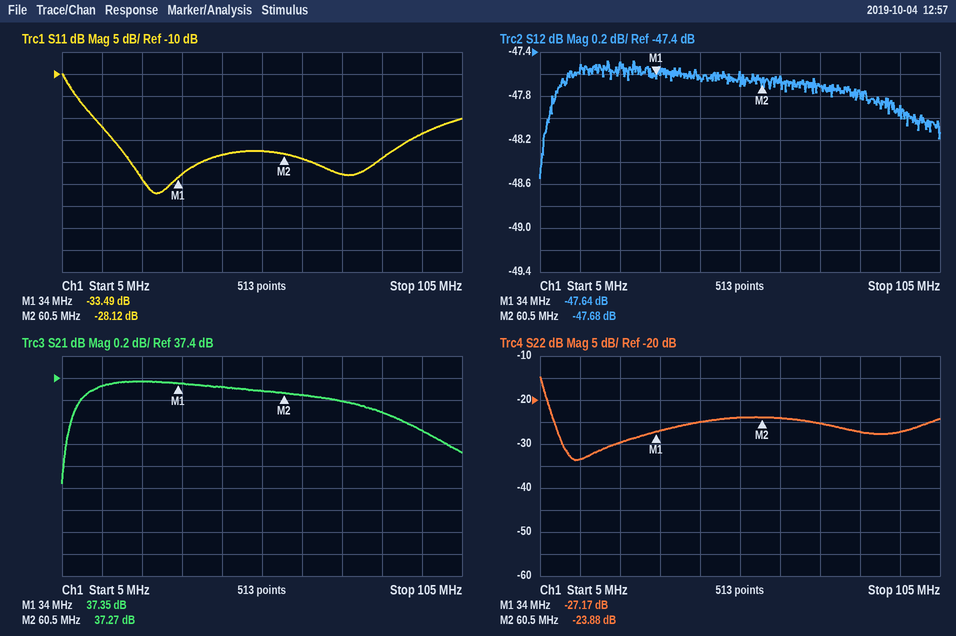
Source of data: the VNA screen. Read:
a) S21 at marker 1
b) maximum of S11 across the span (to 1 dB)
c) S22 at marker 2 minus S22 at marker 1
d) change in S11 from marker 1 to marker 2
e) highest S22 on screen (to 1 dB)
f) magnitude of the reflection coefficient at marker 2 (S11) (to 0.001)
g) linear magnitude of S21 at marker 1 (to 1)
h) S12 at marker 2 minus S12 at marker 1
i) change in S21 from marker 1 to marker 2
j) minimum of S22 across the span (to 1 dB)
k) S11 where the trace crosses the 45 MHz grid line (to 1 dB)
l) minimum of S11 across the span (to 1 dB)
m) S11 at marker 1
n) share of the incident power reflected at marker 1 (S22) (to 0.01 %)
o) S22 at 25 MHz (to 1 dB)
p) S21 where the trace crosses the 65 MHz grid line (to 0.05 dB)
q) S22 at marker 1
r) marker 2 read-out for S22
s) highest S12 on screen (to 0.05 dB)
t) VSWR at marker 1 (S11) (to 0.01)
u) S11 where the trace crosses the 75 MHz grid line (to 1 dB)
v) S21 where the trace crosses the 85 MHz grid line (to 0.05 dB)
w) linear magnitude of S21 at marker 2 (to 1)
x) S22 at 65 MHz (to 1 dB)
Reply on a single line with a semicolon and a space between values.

37.35 dB; -10 dB; 3.29 dB; 5.37 dB; -15 dB; 0.039; 74; -0.04 dB; -0.08 dB; -34 dB; -28 dB; -37 dB; -33.49 dB; 0.19 %; -30 dB; 37.25 dB; -27.17 dB; -23.88 dB; -47.50 dB; 1.04; -33 dB; 37.10 dB; 73; -24 dB
